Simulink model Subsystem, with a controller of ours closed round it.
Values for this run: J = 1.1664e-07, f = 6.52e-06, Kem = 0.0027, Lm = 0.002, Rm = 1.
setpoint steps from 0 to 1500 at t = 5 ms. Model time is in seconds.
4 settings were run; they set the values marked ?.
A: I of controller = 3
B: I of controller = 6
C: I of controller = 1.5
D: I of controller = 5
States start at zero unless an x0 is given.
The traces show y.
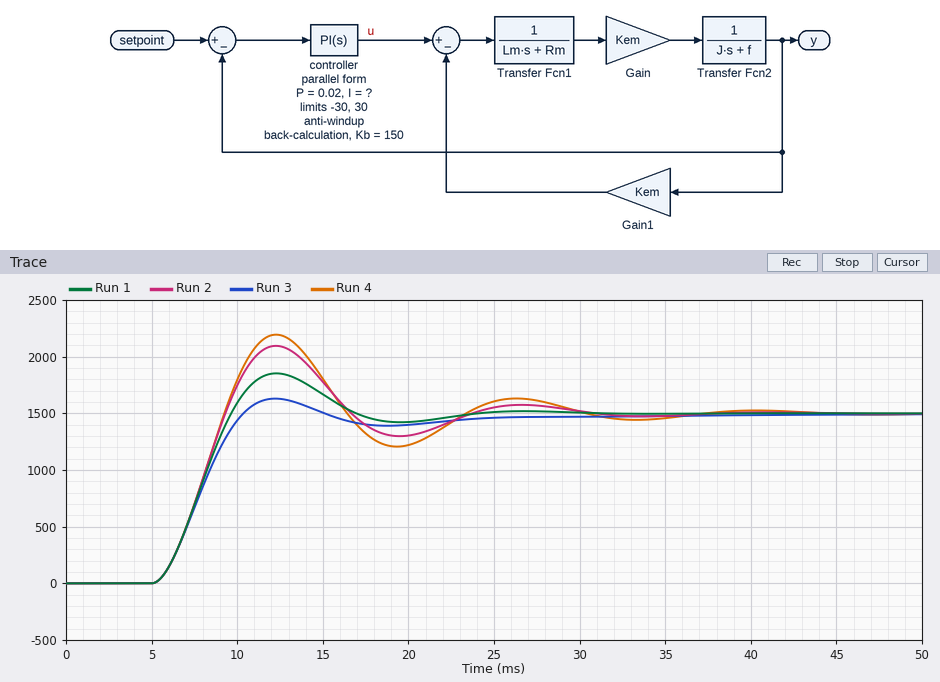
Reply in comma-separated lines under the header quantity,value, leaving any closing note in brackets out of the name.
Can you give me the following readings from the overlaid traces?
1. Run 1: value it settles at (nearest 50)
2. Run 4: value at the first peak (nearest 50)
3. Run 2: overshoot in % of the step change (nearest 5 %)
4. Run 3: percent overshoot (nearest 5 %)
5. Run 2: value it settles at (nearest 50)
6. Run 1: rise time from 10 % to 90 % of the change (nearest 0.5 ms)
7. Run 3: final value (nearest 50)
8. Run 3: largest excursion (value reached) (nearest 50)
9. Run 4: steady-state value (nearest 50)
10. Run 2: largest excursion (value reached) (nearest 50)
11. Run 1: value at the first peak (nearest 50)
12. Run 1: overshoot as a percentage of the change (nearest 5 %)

quantity,value
Run 1: value it settles at,1500
Run 4: value at the first peak,2200
Run 2: overshoot in % of the step change,40 %
Run 3: percent overshoot,10 %
Run 2: value it settles at,1500
Run 1: rise time from 10 % to 90 % of the change,3.0 ms
Run 3: final value,1500
Run 3: largest excursion (value reached),1650
Run 4: steady-state value,1500
Run 2: largest excursion (value reached),2100
Run 1: value at the first peak,1850
Run 1: overshoot as a percentage of the change,25 %
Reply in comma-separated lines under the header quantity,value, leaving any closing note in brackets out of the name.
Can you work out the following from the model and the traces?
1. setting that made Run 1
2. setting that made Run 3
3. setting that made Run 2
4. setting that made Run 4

quantity,value
setting that made Run 1,A
setting that made Run 3,C
setting that made Run 2,D
setting that made Run 4,B
